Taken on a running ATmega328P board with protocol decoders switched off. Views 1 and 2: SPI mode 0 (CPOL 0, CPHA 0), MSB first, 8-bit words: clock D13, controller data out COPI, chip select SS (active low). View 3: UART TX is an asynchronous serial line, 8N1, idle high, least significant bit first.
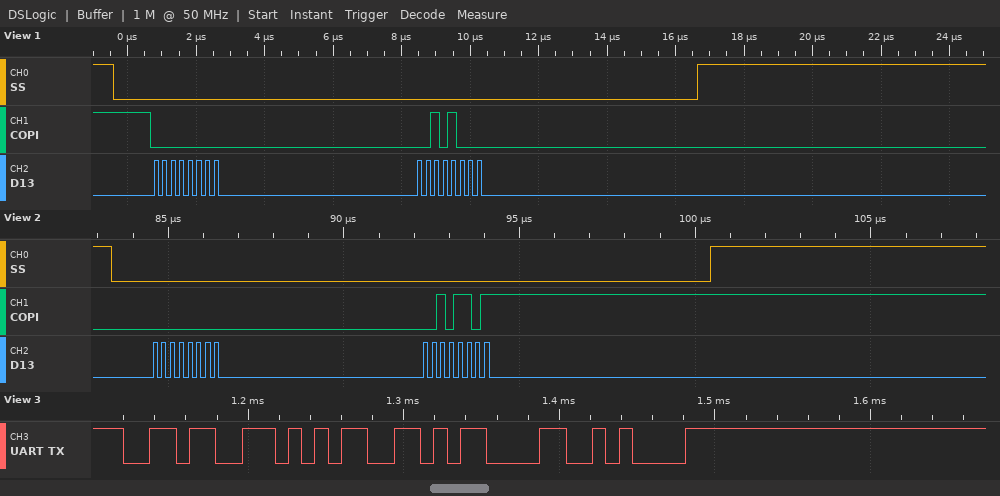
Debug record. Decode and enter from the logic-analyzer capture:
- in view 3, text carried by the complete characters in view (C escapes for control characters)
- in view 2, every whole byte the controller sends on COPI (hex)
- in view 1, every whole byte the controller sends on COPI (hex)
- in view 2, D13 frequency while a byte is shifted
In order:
"65\r\n"
00 2D
0x00 0x28
4 MHz
